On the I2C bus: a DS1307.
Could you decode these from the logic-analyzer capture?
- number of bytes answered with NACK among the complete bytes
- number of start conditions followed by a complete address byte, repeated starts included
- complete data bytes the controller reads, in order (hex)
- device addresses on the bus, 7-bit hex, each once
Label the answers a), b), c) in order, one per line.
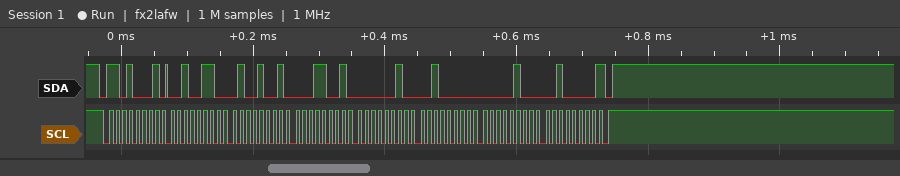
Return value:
a) 1
b) 1
c) 26 49 19 02 20 04 20
d) 0x68
